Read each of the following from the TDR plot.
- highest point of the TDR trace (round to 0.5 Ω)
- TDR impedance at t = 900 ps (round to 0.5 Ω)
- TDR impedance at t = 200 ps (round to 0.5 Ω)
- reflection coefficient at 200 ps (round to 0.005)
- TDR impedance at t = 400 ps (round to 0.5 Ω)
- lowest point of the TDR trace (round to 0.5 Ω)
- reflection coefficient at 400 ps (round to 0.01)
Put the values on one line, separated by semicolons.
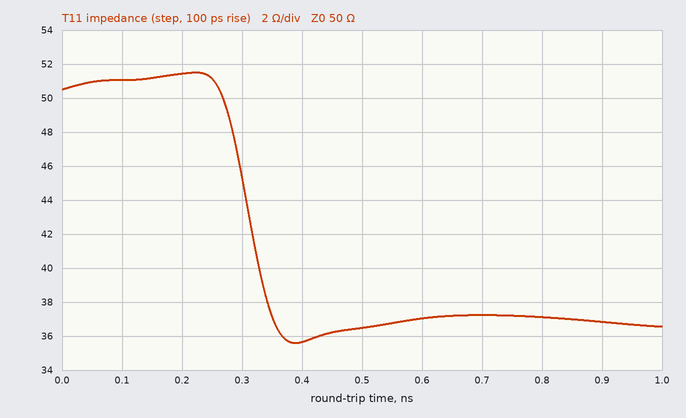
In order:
51.5 Ω; 37.0 Ω; 51.5 Ω; +0.015; 35.5 Ω; 35.5 Ω; -0.17
